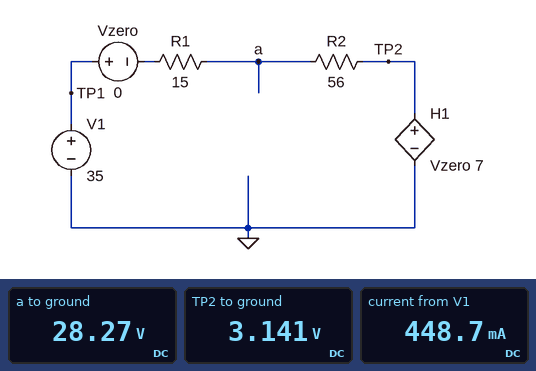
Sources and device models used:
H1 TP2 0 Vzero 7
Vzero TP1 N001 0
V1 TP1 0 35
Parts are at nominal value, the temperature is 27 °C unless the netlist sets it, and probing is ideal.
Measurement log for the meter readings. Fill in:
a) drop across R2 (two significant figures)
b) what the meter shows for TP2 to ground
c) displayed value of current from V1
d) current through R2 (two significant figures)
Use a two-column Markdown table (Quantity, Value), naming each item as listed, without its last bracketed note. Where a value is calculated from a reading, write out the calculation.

| Quantity | Value |
|---|---|
| drop across R2 | 28.27 V - 3.141 V = 25 V |
| what the meter shows for TP2 to ground | 3.141 V |
| displayed value of current from V1 | 448.7 mA |
| current through R2 | (28.27 V - 3.141 V) / 56 Ω = 450 mA |
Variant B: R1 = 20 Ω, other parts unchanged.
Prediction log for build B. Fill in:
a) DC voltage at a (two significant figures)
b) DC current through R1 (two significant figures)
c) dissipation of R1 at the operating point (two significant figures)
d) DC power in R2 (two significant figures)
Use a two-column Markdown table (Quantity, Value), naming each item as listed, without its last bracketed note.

| Quantity | Value |
|---|---|
| DC voltage at a | 27 V |
| DC current through R1 | 420 mA |
| dissipation of R1 at the operating point | 3.6 W |
| DC power in R2 | 10 W |
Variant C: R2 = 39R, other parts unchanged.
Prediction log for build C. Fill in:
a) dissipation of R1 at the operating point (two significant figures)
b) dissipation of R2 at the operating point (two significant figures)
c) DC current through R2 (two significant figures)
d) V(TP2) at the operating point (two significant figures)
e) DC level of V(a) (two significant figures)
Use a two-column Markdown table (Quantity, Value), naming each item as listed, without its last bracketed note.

| Quantity | Value |
|---|---|
| dissipation of R1 at the operating point | 4.9 W |
| dissipation of R2 at the operating point | 13 W |
| DC current through R2 | 570 mA |
| V(TP2) at the operating point | 4.0 V |
| DC level of V(a) | 26 V |
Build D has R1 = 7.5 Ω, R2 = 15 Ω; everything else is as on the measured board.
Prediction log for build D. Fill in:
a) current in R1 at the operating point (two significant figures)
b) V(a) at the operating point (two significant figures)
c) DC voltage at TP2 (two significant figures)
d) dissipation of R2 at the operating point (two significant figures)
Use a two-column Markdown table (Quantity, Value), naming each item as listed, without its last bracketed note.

| Quantity | Value |
|---|---|
| current in R1 at the operating point | 1.2 A |
| V(a) at the operating point | 26 V |
| DC voltage at TP2 | 8.3 V |
| dissipation of R2 at the operating point | 21 W |
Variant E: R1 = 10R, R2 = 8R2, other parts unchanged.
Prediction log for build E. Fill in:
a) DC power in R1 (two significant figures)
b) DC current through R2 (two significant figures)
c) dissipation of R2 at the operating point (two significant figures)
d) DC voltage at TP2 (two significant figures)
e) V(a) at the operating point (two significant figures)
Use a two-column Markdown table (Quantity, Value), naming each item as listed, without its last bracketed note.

| Quantity | Value |
|---|---|
| DC power in R1 | 19 W |
| DC current through R2 | 1.4 A |
| dissipation of R2 at the operating point | 16 W |
| DC voltage at TP2 | 9.7 V |
| V(a) at the operating point | 21 V |
